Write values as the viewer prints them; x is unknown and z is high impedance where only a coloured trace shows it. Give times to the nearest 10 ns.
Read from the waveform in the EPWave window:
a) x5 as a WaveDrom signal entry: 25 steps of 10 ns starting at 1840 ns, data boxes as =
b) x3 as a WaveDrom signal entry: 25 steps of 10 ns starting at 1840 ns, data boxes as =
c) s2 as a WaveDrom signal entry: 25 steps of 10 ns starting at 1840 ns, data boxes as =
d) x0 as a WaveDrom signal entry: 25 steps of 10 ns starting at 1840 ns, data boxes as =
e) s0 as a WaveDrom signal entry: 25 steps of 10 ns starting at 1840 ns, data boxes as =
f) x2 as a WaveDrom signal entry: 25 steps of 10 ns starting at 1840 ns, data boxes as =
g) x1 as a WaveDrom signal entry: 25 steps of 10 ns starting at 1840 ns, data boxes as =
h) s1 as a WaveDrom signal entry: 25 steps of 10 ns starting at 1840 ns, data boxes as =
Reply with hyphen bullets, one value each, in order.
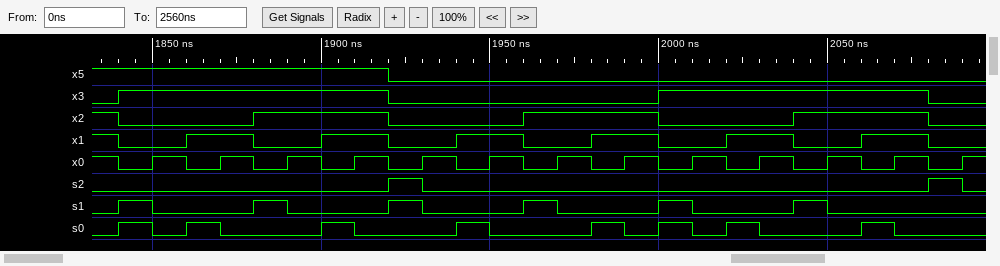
- {name: 'x5', wave: '1.......0................'}
- {name: 'x3', wave: '1.......0.......1.......0'}
- {name: 's2', wave: '0.......10..............1'}
- {name: 'x0', wave: '0101010101010101010101010'}
- {name: 's0', wave: '1010..10..10..101010..10.'}
- {name: 'x2', wave: '0...1...0...1...0...1...0'}
- {name: 'x1', wave: '0.1.0.1.0.1.0.1.0.1.0.1.0'}
- {name: 's1', wave: '10..10..10..10..10..10...'}
